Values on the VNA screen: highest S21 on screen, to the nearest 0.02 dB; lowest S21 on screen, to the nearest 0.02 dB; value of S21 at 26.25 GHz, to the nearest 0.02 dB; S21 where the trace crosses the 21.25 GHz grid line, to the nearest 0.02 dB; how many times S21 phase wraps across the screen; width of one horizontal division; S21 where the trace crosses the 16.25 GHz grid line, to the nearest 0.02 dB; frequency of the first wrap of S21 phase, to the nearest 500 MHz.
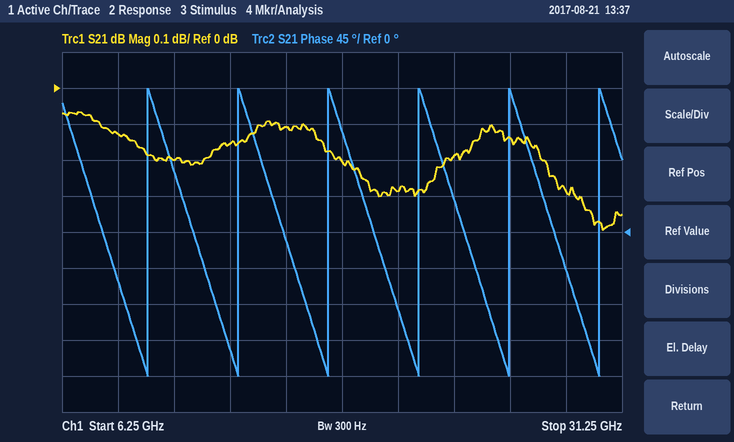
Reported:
-0.06 dB
-0.40 dB
-0.14 dB
-0.28 dB
6
2.5 GHz
-0.10 dB
10.0 GHz
